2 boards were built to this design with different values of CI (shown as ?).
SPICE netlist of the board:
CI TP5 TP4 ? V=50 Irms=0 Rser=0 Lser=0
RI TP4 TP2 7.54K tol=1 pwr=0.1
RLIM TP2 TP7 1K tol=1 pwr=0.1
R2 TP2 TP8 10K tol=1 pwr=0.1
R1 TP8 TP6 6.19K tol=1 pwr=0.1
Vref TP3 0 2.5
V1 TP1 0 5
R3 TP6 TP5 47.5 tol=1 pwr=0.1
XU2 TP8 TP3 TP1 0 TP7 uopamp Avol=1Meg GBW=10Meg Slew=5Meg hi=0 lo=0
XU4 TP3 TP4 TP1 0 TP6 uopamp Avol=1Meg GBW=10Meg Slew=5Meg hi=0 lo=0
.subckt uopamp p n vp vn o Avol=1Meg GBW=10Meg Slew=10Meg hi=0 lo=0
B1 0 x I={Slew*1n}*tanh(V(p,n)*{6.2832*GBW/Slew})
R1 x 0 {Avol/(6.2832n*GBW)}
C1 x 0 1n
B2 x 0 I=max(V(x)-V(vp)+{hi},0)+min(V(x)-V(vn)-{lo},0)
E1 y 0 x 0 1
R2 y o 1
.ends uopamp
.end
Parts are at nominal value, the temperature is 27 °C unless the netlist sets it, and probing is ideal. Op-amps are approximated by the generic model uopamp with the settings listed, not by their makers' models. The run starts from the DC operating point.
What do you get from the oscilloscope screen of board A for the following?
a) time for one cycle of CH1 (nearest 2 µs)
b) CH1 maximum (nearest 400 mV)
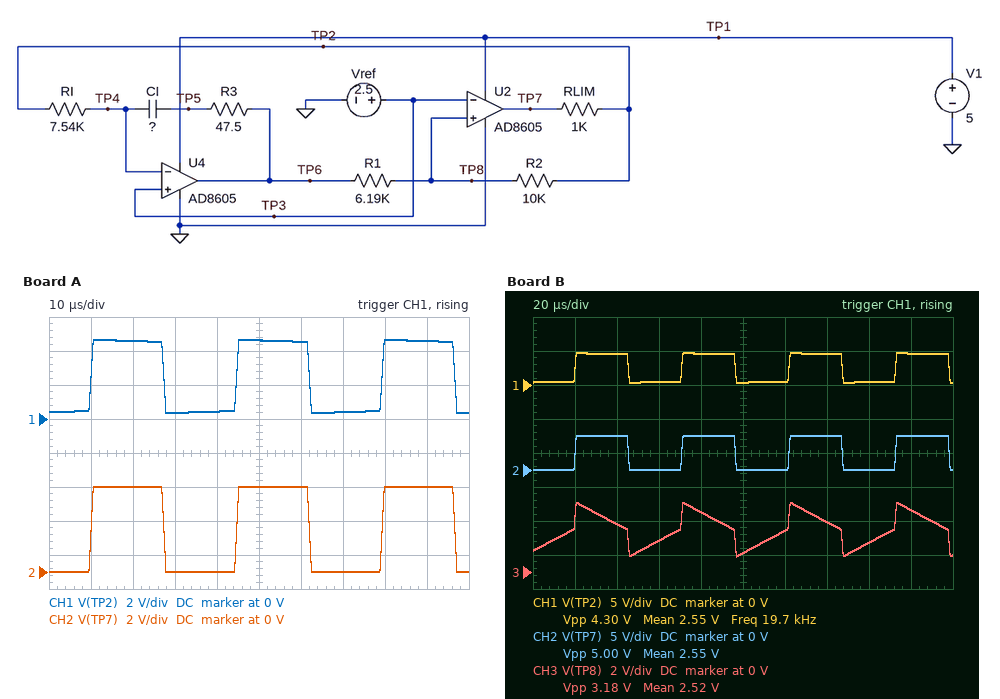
34 µs
4.8 V
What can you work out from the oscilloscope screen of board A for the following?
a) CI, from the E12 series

1.8 nF
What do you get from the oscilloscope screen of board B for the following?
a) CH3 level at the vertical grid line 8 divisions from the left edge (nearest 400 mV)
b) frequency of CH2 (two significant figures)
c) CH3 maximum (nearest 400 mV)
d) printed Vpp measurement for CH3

1.6 V
20 kHz
4.0 V
3.18 V
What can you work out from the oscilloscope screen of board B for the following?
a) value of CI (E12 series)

2.7 nF
